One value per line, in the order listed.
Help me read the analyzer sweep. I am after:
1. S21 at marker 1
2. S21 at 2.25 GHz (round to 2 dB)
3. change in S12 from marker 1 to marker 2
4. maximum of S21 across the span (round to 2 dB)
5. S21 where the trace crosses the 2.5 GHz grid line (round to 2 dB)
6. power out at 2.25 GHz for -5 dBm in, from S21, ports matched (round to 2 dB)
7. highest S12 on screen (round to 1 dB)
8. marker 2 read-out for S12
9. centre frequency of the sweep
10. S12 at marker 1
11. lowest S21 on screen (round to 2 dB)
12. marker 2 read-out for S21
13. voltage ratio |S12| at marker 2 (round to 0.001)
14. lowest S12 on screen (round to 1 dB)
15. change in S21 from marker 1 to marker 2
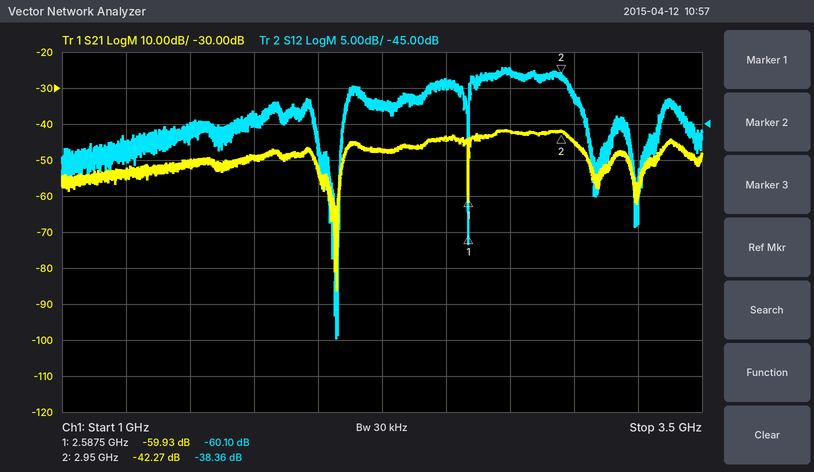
-59.93 dB
-48 dB
21.74 dB
-42 dB
-44 dB
-52 dBm
-37 dB
-38.36 dB
2.25 GHz
-60.10 dB
-86 dB
-42.27 dB
0.012
-75 dB
17.66 dB
